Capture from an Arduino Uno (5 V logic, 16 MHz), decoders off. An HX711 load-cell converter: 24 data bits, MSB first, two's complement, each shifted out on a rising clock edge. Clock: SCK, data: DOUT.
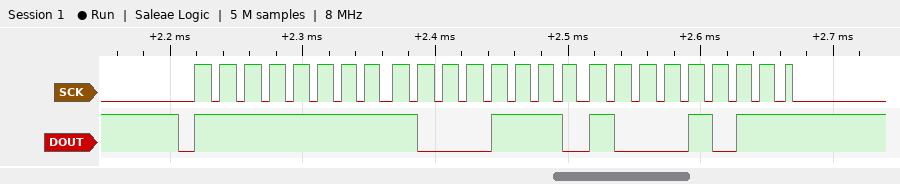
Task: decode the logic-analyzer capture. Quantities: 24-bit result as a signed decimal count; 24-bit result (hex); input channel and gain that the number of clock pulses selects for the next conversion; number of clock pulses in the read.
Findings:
-29045
0xFF8E8B
channel A, gain 128
25
